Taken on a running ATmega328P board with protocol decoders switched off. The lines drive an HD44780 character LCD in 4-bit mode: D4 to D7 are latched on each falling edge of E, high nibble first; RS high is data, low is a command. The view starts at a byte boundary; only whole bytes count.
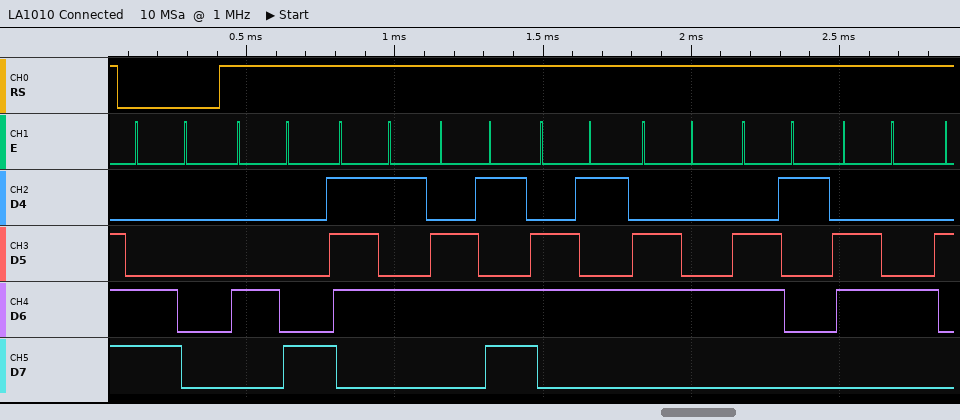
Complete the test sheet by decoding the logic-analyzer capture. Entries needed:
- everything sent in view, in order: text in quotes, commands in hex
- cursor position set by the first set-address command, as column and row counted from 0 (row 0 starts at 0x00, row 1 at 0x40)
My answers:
0xC0 "Humedad"
column 0, row 1
